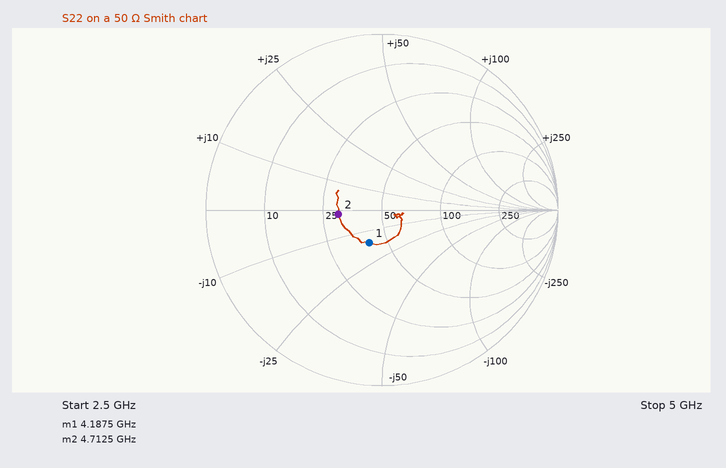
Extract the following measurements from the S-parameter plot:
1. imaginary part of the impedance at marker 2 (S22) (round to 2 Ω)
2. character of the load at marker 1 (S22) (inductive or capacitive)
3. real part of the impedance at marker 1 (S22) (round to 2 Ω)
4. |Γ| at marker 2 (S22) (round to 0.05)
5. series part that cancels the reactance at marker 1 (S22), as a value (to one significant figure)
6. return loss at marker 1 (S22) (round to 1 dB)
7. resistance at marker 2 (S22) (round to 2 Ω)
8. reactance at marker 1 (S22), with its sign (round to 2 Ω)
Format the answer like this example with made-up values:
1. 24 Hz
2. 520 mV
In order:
1. -2 Ω
2. capacitive
3. 40 Ω
4. 0.25
5. 600 pH
6. 14 dB
7. 30 Ω
8. -16 Ω
